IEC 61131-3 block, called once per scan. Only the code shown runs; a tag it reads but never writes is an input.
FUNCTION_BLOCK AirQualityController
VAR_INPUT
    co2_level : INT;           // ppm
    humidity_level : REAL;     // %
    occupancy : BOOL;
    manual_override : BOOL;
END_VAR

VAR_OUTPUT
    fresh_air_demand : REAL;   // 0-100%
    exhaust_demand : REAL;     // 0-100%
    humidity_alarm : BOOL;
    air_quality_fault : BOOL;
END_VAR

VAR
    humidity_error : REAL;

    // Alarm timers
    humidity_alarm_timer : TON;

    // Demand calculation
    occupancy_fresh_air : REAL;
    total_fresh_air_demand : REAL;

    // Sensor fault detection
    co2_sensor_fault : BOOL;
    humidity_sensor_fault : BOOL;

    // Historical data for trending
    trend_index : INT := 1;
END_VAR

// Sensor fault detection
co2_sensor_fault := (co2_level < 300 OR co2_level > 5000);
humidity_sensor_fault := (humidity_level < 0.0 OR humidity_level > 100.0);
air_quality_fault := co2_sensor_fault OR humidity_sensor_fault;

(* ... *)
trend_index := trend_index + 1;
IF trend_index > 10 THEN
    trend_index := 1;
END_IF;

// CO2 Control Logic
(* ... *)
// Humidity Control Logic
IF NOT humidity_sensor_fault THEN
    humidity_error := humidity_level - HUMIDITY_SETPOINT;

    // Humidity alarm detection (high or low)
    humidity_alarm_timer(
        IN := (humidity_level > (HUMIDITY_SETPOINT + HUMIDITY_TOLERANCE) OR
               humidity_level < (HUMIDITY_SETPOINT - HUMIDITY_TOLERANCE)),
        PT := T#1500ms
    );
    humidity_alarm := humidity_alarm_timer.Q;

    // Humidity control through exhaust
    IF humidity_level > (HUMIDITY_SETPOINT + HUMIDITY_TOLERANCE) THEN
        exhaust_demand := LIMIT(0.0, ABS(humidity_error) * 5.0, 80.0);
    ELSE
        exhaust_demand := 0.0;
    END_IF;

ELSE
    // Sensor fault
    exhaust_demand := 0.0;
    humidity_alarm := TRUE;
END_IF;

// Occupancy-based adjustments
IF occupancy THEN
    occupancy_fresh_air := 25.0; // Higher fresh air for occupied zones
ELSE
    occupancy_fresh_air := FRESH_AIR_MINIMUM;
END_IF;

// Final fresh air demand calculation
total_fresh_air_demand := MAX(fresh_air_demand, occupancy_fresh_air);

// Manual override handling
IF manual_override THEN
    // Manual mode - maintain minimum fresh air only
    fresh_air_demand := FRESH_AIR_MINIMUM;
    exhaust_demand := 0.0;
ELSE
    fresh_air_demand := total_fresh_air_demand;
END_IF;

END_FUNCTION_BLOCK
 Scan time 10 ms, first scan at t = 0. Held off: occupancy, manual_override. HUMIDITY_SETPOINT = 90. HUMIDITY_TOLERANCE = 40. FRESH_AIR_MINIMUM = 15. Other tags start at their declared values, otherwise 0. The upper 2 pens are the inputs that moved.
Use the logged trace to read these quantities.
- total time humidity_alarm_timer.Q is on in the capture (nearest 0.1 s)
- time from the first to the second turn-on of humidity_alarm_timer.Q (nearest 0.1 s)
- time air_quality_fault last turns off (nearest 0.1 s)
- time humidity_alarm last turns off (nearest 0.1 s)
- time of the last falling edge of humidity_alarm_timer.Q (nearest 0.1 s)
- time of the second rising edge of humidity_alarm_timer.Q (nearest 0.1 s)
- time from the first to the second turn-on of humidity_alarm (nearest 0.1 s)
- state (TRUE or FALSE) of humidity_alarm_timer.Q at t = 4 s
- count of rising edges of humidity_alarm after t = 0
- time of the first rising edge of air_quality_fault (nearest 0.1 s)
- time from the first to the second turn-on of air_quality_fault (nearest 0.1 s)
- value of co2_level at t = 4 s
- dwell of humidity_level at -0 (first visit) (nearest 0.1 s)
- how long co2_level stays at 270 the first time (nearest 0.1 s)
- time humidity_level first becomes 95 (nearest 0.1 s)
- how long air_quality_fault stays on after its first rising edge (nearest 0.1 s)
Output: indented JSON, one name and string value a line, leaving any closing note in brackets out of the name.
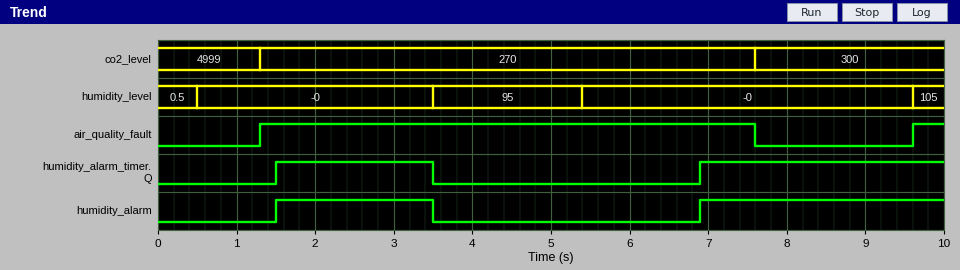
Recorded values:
{
  "total time humidity_alarm_timer.Q is on in the capture": "5.1 s",
  "time from the first to the second turn-on of humidity_alarm_timer.Q": "5.4 s",
  "time air_quality_fault last turns off": "7.6 s",
  "time humidity_alarm last turns off": "3.5 s",
  "time of the last falling edge of humidity_alarm_timer.Q": "3.5 s",
  "time of the second rising edge of humidity_alarm_timer.Q": "6.9 s",
  "time from the first to the second turn-on of humidity_alarm": "5.4 s",
  "state (TRUE or FALSE) of humidity_alarm_timer.Q at t = 4 s": "FALSE",
  "count of rising edges of humidity_alarm after t = 0": "2",
  "time of the first rising edge of air_quality_fault": "1.3 s",
  "time from the first to the second turn-on of air_quality_fault": "8.3 s",
  "value of co2_level at t = 4 s": "270",
  "dwell of humidity_level at -0 (first visit)": "3.0 s",
  "how long co2_level stays at 270 the first time": "6.3 s",
  "time humidity_level first becomes 95": "3.5 s",
  "how long air_quality_fault stays on after its first rising edge": "6.3 s"
}
